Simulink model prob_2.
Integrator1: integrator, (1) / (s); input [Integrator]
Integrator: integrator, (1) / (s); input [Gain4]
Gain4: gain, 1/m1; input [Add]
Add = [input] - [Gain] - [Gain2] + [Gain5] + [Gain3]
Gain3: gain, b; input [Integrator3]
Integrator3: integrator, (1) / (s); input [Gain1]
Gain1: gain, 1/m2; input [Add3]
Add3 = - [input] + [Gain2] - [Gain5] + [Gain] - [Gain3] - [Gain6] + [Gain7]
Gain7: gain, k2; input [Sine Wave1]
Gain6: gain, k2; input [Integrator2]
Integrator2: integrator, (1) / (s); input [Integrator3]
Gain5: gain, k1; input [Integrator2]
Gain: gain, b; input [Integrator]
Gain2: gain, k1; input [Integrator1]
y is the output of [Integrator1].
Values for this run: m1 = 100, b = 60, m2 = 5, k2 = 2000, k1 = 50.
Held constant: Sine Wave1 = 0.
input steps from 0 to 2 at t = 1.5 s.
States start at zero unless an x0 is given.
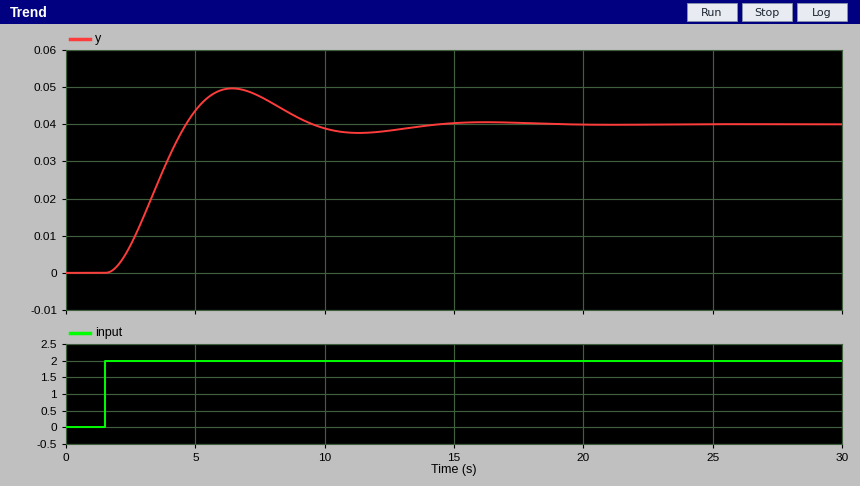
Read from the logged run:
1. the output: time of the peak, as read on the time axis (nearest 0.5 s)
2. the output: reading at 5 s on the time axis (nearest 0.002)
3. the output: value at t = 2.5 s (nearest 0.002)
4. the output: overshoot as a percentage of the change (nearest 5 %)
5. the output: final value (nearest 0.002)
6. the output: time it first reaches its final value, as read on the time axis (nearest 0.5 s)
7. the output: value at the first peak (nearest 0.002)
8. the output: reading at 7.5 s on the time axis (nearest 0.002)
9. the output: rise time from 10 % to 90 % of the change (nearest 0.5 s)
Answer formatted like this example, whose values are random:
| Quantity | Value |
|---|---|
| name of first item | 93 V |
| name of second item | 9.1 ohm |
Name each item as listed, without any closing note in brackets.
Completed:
| Quantity | Value |
|---|---|
| the output: time of the peak, as read on the time axis | 6.5 s |
| the output: reading at 5 s on the time axis | 0.044 |
| the output: value at t = 2.5 s | 0.008 |
| the output: overshoot as a percentage of the change | 25 % |
| the output: final value | 0.040 |
| the output: time it first reaches its final value, as read on the time axis | 4.5 s |
| the output: value at the first peak | 0.050 |
| the output: reading at 7.5 s on the time axis | 0.048 |
| the output: rise time from 10 % to 90 % of the change | 2.0 s |
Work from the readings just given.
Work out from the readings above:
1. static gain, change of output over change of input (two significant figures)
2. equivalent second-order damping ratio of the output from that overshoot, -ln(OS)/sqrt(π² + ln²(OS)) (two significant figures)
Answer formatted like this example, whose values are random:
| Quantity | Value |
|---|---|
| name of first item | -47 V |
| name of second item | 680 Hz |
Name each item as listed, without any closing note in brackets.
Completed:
| Quantity | Value |
|---|---|
| static gain, change of output over change of input | 0.020 |
| equivalent second-order damping ratio of the output from that overshoot, -ln(OS)/sqrt(π² + ln²(OS)) | 0.40 |
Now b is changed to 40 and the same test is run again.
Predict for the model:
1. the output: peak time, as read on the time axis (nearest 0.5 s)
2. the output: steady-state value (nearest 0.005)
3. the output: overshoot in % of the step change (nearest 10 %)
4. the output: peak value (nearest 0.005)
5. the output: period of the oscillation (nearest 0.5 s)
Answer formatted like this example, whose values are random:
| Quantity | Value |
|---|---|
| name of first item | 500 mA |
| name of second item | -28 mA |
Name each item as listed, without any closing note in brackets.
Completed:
| Quantity | Value |
|---|---|
| the output: peak time, as read on the time axis | 6.0 s |
| the output: steady-state value | 0.040 |
| the output: overshoot in % of the step change | 40 % |
| the output: peak value | 0.055 |
| the output: period of the oscillation | 9.5 s |
